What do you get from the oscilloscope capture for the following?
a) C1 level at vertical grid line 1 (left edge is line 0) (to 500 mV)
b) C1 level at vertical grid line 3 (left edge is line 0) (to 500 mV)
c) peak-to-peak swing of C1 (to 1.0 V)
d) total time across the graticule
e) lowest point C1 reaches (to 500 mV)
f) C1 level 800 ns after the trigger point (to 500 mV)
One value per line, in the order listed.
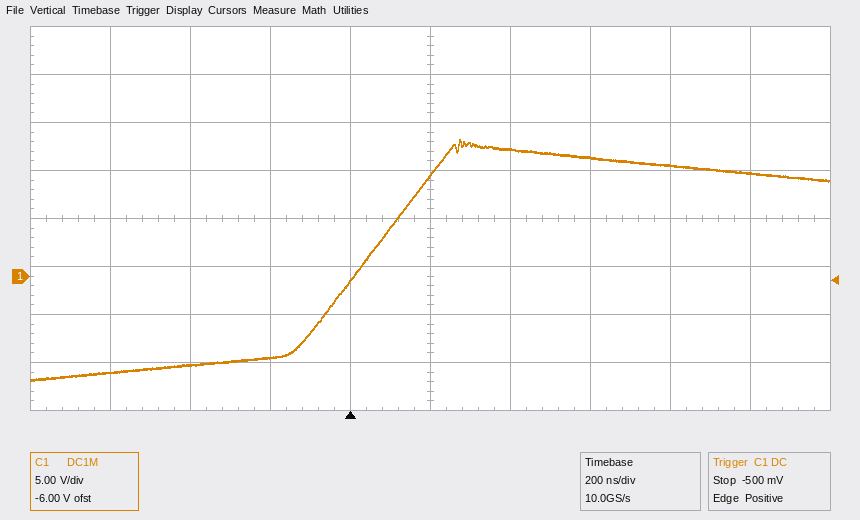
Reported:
-10.0 V
-8.5 V
25.0 V
2 µs
-11.0 V
11.5 V
